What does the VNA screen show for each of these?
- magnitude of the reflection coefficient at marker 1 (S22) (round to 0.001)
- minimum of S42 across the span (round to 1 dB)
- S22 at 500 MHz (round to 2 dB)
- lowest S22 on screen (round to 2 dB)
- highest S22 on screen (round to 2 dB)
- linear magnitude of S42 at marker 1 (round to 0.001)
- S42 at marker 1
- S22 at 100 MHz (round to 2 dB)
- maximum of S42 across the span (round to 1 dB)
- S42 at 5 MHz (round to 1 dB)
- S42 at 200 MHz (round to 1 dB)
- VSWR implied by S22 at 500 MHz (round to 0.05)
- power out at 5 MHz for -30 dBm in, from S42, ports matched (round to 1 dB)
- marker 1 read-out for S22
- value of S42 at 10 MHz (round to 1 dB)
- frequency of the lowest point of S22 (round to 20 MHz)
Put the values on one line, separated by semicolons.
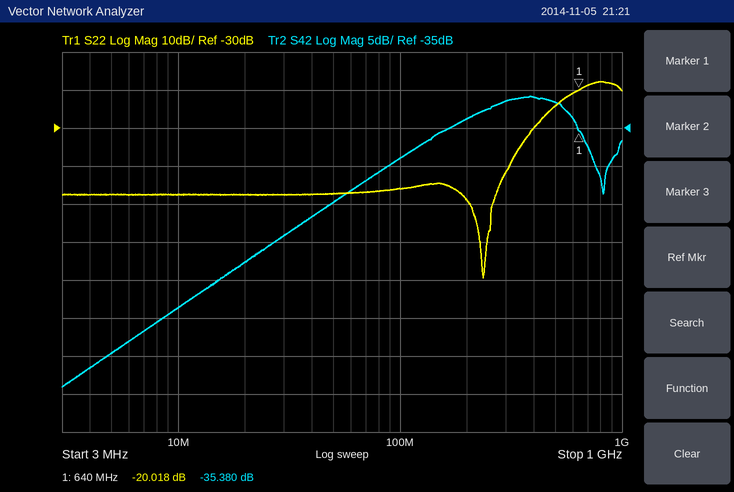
0.100; -69 dB; -24 dB; -70 dB; -18 dB; 0.017; -35.380 dB; -46 dB; -31 dB; -65 dB; -34 dB; 1.15; -95 dBm; -20.018 dB; -59 dB; 240 MHz
